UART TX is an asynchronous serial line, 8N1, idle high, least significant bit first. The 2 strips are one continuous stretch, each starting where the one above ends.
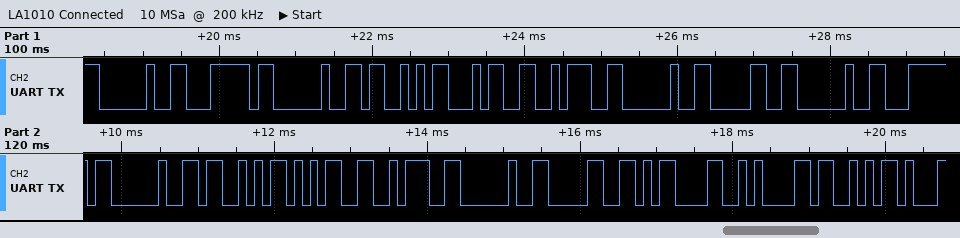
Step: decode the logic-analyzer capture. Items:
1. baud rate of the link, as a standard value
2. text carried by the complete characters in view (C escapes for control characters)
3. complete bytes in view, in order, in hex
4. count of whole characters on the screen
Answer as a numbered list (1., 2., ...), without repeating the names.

1. 9600 baud
2. " | S4: 0 | S5: 0\r\nS"
3. 20 7C 20 53 34 3A 20 30 20 7C 20 53 35 3A 20 30 0D 0A 53
4. 19
